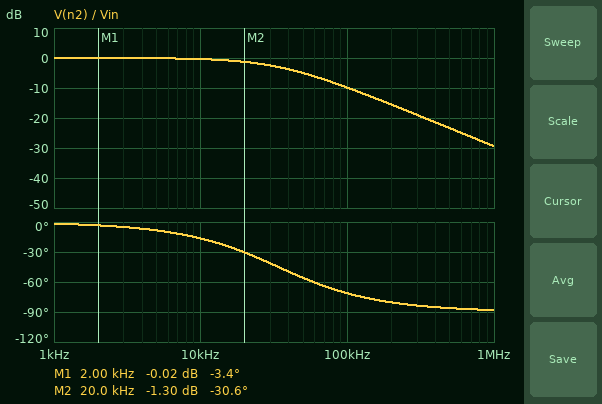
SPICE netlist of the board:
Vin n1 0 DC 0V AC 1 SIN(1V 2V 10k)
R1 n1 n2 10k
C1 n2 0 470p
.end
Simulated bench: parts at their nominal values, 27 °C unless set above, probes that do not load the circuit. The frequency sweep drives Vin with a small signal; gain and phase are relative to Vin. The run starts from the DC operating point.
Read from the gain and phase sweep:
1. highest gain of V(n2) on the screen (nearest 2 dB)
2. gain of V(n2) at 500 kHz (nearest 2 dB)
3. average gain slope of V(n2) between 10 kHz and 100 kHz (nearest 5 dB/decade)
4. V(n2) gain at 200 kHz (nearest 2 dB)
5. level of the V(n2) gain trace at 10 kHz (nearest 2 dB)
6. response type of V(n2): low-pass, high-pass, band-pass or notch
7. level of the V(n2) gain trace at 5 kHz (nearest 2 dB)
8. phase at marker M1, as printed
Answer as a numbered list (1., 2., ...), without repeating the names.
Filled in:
1. 0 dB
2. -24 dB
3. -10 dB/decade
4. -16 dB
5. 0 dB
6. low-pass
7. 0 dB
8. -3.4 deg
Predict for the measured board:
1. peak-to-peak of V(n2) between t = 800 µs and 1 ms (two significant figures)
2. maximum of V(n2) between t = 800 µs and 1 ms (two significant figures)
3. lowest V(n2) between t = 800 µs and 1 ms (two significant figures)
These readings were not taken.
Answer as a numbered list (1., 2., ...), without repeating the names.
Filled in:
1. 3.8 V
2. 2.9 V
3. -920 mV
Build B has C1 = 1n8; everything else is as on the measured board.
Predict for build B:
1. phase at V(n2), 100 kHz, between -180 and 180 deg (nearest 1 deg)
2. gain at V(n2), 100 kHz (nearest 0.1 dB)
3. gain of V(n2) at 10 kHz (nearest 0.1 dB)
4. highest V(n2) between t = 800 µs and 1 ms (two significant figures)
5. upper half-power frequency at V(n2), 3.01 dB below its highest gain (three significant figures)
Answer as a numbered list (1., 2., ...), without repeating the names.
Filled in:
1. -85 deg
2. -21.1 dB
3. -3.6 dB
4. 2.3 V
5. 8.84 kHz
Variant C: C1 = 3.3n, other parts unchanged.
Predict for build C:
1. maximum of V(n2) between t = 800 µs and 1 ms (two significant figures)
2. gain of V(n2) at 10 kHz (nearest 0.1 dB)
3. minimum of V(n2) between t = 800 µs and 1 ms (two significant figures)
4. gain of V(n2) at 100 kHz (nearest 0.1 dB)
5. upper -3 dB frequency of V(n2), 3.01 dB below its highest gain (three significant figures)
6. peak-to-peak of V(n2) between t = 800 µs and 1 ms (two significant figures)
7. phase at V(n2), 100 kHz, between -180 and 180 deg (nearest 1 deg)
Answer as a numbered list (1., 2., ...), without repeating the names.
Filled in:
1. 1.9 V
2. -7.2 dB
3. 130 mV
4. -26.3 dB
5. 4.82 kHz
6. 1.7 V
7. -87 deg
